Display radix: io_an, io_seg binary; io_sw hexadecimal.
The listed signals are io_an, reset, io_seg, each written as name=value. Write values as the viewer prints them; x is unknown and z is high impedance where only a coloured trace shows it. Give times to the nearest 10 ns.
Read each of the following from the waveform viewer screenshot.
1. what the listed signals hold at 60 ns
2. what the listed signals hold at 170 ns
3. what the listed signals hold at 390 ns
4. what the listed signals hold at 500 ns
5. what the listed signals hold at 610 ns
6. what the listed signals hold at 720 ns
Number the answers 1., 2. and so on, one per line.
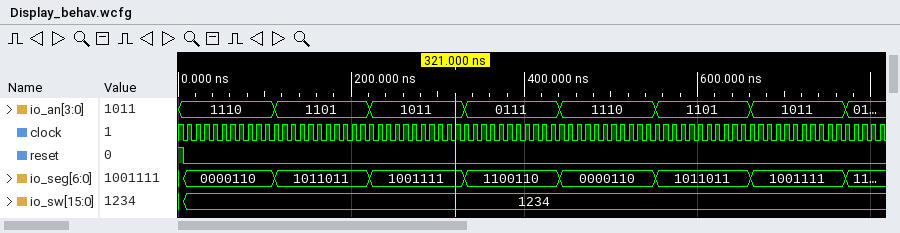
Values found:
1. io_an=1110, reset=0, io_seg=0000110
2. io_an=1101, reset=0, io_seg=1011011
3. io_an=0111, reset=0, io_seg=1100110
4. io_an=1110, reset=0, io_seg=0000110
5. io_an=1101, reset=0, io_seg=1011011
6. io_an=1011, reset=0, io_seg=1001111
